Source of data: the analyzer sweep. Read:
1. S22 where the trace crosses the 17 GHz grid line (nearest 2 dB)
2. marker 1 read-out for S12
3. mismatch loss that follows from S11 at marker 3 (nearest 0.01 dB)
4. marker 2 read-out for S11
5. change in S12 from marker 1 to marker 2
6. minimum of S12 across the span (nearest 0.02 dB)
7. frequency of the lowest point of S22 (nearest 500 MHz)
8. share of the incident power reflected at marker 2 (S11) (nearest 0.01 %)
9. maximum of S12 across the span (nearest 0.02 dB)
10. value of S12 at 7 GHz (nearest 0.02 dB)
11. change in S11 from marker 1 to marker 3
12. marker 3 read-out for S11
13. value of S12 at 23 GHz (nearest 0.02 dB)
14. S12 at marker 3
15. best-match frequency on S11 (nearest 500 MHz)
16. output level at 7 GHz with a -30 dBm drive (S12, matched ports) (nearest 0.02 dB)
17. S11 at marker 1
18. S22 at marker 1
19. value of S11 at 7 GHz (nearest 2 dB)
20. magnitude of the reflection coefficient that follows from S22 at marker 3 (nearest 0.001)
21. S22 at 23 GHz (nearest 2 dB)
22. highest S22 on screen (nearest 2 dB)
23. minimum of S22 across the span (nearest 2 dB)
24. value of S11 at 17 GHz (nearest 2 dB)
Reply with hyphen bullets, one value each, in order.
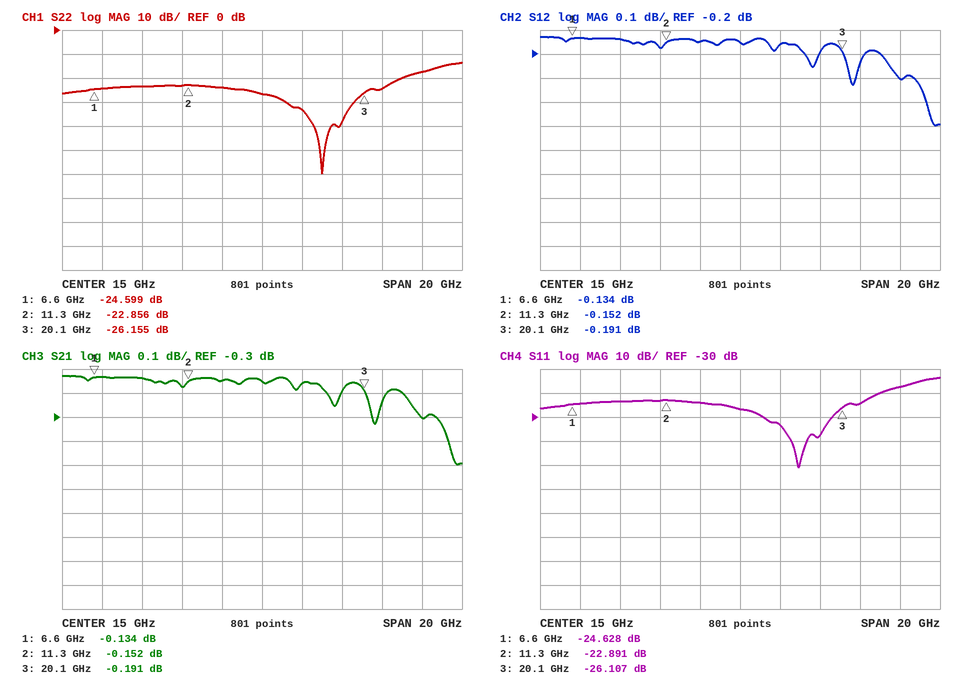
- -34 dB
- -0.134 dB
- 0.01 dB
- -22.891 dB
- -0.018 dB
- -0.50 dB
- 18.0 GHz
- 0.51 %
- -0.12 dB
- -0.14 dB
- -1.479 dB
- -26.107 dB
- -0.30 dB
- -0.191 dB
- 18.0 GHz
- -30.14 dBm
- -24.628 dB
- -24.599 dB
- -24 dB
- 0.049
- -18 dB
- -14 dB
- -60 dB
- -34 dB
